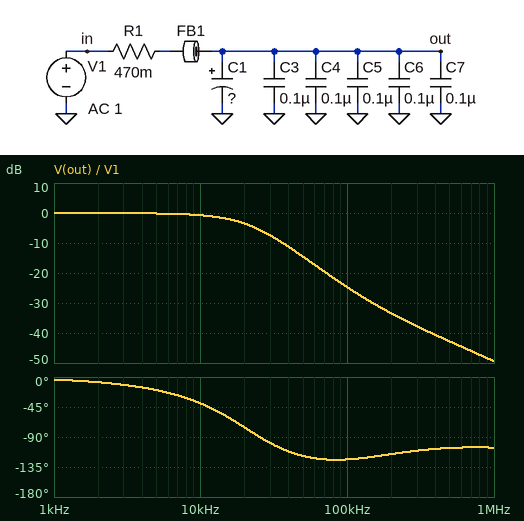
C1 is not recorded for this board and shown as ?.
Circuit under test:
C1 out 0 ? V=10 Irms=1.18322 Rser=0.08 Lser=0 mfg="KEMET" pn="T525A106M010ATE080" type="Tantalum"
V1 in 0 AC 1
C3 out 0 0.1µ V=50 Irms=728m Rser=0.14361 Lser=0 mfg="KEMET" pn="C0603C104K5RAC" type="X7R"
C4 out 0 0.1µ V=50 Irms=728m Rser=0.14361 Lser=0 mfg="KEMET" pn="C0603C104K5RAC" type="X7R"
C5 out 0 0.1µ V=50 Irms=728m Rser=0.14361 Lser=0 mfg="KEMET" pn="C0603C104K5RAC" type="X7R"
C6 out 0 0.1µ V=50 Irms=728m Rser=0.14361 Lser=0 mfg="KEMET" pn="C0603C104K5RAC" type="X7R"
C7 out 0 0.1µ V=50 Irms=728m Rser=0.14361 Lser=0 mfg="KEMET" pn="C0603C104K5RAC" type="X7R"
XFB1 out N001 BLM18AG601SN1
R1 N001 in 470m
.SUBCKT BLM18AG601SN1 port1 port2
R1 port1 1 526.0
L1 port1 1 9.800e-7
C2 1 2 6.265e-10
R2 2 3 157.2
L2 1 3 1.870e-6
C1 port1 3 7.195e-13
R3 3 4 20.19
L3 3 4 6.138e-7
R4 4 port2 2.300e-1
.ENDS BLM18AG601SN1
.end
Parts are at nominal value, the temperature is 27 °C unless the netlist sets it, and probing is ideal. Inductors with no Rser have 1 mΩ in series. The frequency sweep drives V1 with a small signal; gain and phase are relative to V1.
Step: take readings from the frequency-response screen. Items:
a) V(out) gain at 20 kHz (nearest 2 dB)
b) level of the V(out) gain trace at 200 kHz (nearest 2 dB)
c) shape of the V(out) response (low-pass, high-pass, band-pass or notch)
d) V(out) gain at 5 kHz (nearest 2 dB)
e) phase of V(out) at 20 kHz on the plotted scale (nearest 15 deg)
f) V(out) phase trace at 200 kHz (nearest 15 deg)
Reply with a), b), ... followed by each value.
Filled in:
a) -4 dB
b) -34 dB
c) low-pass
d) 0 dB
e) -75 deg
f) -120 deg
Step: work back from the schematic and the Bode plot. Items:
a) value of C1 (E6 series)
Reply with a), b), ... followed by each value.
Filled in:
a) 15 µF
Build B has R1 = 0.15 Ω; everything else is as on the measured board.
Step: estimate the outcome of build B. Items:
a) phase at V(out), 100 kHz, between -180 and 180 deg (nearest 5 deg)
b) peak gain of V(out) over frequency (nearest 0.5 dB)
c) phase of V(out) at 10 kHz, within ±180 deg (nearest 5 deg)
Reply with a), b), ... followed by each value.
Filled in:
a) -130 deg
b) 1.5 dB
c) -25 deg
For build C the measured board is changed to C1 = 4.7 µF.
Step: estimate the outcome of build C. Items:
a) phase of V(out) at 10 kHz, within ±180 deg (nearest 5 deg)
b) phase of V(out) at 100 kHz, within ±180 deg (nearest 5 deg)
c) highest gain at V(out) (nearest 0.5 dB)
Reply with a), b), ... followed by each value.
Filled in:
a) -15 deg
b) -145 deg
c) 1.5 dB
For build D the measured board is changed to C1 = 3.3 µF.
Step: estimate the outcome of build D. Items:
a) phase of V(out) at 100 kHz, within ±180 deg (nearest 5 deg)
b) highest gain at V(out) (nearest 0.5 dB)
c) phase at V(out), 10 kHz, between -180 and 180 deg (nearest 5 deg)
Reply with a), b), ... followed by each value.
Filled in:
a) -150 deg
b) 2.5 dB
c) -10 deg
